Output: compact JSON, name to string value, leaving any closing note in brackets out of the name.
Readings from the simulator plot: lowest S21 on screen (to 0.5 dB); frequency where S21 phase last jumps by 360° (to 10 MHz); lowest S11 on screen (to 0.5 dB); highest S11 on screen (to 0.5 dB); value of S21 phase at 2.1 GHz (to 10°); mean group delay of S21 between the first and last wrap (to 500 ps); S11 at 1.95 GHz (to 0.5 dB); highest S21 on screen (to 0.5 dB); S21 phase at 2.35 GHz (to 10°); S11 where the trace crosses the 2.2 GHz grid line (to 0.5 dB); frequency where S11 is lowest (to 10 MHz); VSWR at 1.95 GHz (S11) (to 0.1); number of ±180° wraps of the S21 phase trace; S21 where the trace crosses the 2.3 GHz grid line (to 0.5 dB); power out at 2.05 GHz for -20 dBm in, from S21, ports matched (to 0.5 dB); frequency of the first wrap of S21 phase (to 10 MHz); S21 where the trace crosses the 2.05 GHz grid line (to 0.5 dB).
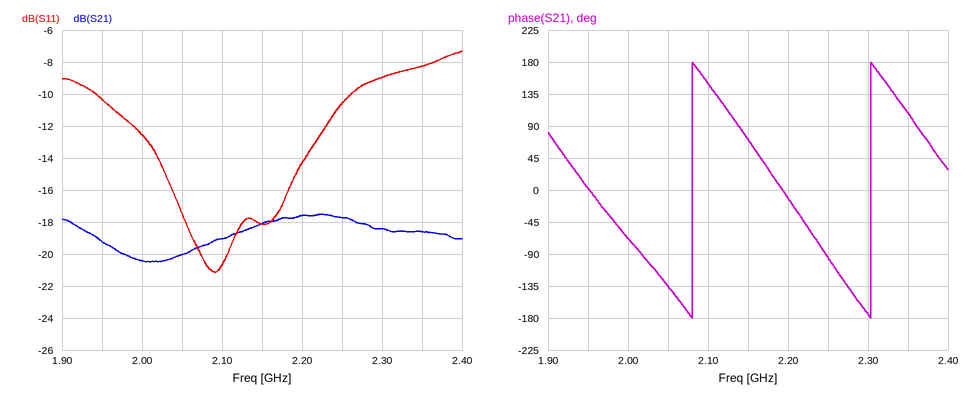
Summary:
{"lowest S21 on screen": "-20.5 dB", "frequency where S21 phase last jumps by 360°": "2.30 GHz", "lowest S11 on screen": "-21.0 dB", "highest S11 on screen": "-7.5 dB", "value of S21 phase at 2.1 GHz": "150°", "mean group delay of S21 between the first and last wrap": "4.5 ns", "S11 at 1.95 GHz": "-10.5 dB", "highest S21 on screen": "-17.5 dB", "S21 phase at 2.35 GHz": "110°", "S11 where the trace crosses the 2.2 GHz grid line": "-14.5 dB", "frequency where S11 is lowest": "2.09 GHz", "VSWR at 1.95 GHz (S11)": "1.9", "number of ±180° wraps of the S21 phase trace": "2", "S21 where the trace crosses the 2.3 GHz grid line": "-18.5 dB", "power out at 2.05 GHz for -20 dBm in, from S21, ports matched": "-40.0 dBm", "frequency of the first wrap of S21 phase": "2.08 GHz", "S21 where the trace crosses the 2.05 GHz grid line": "-20.0 dB"}
